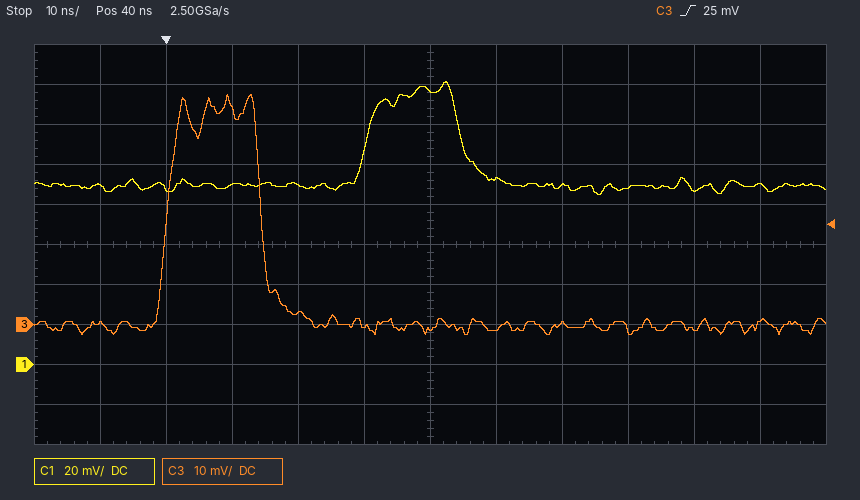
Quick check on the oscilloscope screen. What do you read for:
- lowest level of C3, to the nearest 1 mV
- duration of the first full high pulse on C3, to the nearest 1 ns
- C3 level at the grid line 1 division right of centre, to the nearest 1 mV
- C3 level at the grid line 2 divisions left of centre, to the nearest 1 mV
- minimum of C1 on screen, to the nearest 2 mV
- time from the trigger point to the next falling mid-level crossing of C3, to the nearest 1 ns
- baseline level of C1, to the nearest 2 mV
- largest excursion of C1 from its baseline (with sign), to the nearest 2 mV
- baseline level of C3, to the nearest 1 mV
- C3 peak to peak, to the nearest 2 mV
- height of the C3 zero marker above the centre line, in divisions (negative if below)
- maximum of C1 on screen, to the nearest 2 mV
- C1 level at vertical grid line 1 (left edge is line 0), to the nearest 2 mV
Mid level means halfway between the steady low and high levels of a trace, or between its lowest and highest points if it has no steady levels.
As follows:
-2 mV
14 ns
-1 mV
3 mV
84 mV
14 ns
90 mV
+52 mV
0 mV
60 mV
-2.0 div
142 mV
90 mV
